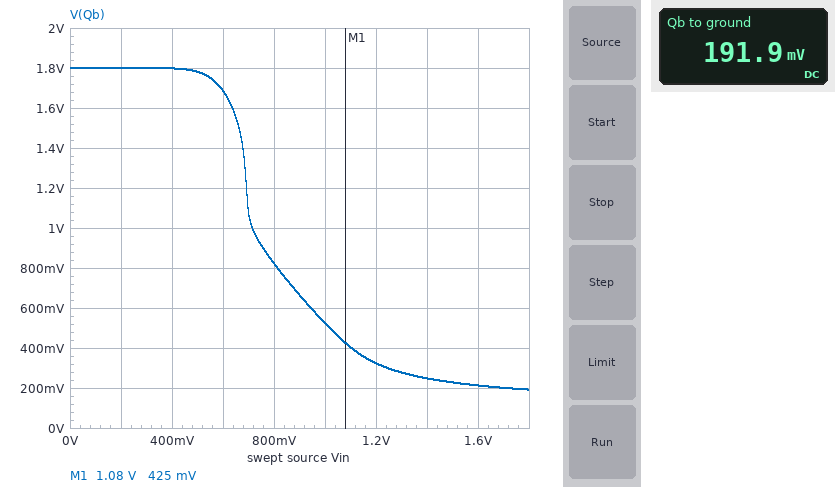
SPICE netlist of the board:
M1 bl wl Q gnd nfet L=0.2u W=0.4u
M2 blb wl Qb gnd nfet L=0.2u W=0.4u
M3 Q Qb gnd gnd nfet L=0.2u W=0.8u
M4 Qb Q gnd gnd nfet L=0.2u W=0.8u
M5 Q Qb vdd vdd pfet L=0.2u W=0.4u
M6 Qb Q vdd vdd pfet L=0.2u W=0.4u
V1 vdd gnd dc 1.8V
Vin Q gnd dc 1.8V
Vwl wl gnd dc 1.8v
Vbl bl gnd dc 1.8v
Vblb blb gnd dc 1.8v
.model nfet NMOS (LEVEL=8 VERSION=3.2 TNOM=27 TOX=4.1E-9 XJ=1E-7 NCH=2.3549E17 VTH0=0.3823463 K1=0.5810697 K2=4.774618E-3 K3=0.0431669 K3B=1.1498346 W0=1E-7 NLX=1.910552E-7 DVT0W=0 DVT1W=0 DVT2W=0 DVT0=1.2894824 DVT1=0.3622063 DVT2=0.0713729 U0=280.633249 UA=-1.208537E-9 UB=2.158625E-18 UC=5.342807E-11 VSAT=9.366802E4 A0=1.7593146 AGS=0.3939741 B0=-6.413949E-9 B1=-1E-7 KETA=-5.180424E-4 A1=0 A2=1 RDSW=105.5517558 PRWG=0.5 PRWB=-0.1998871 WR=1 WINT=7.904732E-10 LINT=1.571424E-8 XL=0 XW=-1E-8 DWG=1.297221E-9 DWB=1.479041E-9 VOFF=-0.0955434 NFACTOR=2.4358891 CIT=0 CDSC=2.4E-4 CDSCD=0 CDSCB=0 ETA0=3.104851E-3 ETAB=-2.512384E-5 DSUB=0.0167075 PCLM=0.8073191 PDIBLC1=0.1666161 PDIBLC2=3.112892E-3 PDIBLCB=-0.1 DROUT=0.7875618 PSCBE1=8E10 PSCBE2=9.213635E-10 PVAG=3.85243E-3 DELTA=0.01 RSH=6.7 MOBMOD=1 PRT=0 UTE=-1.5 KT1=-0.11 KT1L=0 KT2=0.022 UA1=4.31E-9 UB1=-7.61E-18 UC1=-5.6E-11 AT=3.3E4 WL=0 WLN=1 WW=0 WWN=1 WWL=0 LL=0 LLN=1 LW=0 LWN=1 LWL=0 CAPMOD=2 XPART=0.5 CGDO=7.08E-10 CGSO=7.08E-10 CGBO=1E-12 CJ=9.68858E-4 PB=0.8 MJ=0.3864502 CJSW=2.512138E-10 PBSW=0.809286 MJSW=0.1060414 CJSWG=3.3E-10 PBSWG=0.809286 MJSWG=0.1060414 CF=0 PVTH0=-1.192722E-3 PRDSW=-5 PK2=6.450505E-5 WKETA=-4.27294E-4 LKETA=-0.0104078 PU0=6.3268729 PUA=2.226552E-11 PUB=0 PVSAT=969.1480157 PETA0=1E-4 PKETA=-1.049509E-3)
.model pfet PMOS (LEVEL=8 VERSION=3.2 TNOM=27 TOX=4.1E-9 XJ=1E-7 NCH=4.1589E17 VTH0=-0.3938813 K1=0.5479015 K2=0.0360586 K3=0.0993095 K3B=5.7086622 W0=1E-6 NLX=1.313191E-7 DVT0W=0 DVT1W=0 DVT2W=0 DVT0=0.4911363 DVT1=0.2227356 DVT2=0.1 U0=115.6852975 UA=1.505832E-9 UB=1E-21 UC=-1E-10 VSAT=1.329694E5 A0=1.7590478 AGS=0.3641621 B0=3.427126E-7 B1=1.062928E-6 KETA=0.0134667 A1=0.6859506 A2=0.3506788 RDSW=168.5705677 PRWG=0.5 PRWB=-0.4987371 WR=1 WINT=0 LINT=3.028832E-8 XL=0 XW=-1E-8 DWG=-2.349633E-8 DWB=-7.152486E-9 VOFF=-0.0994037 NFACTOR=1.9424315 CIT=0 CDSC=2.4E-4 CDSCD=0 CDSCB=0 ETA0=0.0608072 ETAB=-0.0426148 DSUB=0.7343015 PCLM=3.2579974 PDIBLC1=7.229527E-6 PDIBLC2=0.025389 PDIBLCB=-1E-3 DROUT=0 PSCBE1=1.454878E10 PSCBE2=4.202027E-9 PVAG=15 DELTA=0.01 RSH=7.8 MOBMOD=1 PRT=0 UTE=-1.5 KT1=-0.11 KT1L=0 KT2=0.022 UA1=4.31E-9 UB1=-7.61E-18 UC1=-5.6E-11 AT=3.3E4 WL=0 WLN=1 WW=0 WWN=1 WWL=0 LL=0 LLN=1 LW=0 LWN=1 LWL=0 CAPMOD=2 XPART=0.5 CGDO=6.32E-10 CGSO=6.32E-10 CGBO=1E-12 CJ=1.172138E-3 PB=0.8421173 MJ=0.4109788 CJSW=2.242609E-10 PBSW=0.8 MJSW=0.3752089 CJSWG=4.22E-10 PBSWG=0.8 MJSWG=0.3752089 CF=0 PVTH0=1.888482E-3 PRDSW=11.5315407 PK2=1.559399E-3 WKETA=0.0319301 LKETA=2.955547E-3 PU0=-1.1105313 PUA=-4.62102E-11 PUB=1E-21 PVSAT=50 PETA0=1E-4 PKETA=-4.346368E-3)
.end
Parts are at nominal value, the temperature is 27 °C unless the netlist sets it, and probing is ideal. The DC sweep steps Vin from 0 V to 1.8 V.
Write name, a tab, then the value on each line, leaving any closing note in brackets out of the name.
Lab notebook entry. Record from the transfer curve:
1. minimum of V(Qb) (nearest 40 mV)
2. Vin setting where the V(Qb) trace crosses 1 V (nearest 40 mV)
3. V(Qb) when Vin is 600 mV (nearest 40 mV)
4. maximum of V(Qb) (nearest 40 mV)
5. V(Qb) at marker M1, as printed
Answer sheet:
minimum of V(Qb)	200 mV
Vin setting where the V(Qb) trace crosses 1 V	720 mV
V(Qb) when Vin is 600 mV	1.68 V
maximum of V(Qb)	1.80 V
V(Qb) at marker M1, as printed	425 mV
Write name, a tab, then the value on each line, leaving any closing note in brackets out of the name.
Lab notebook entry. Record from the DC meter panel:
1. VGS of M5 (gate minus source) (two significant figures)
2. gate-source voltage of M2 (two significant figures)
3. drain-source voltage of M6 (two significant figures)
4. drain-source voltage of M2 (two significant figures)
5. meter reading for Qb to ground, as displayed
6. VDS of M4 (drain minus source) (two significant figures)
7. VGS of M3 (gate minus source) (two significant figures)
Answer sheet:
VGS of M5 (gate minus source)	-1.6 V
gate-source voltage of M2	1.6 V
drain-source voltage of M6	-1.6 V
drain-source voltage of M2	1.6 V
meter reading for Qb to ground, as displayed	191.9 mV
VDS of M4 (drain minus source)	190 mV
VGS of M3 (gate minus source)	190 mV
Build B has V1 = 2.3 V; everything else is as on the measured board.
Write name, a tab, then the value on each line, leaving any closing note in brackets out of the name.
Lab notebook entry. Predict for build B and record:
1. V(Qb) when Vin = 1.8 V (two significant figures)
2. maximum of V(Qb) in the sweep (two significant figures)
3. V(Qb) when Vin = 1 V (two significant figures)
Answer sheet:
V(Qb) when Vin = 1.8 V	190 mV
maximum of V(Qb) in the sweep	2.3 V
V(Qb) when Vin = 1 V	670 mV
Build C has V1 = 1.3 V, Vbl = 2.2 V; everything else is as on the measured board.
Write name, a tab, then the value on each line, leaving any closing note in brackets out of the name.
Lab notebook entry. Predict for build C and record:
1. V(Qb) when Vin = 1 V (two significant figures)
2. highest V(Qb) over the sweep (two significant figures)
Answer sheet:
V(Qb) when Vin = 1 V	490 mV
highest V(Qb) over the sweep	1.3 V
